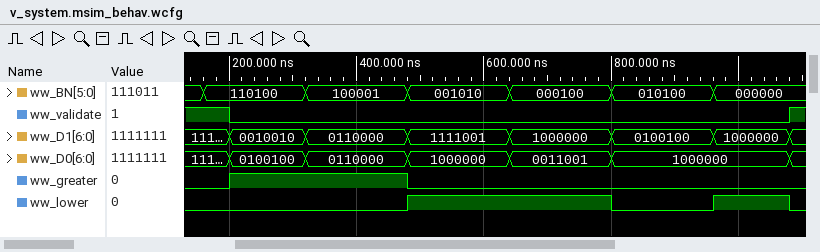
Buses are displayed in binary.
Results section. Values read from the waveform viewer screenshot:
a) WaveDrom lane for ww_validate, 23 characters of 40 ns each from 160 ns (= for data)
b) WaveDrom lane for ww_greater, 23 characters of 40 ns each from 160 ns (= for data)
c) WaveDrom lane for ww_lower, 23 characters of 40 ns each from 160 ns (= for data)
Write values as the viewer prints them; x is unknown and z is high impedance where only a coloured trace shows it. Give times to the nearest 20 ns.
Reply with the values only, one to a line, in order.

{name: 'ww_validate', wave: '10.....................'}
{name: 'ww_greater', wave: '01......0..............'}
{name: 'ww_lower', wave: '0.......1.......0...1..'}
